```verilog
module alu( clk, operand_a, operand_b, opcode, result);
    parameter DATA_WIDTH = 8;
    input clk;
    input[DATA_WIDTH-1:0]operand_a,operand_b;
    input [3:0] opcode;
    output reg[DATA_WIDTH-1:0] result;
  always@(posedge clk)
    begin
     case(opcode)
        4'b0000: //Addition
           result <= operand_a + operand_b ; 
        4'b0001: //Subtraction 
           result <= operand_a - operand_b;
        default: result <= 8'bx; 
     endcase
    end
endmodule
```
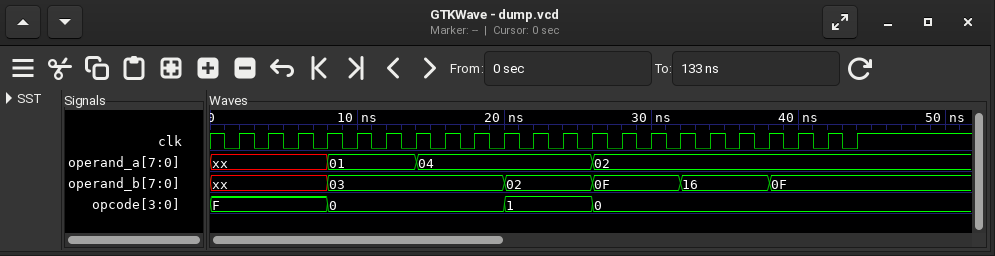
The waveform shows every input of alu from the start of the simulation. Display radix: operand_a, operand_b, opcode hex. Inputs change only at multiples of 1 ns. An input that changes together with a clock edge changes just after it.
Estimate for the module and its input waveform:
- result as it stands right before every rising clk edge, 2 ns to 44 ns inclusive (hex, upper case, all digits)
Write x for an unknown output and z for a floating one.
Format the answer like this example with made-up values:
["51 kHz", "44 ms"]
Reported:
["x, x, x, x, x, 04, 04, 04, 07, 07, 07, 02, 02, 02, 11, 11, 11, 18, 18, 18, 11, 11"]
